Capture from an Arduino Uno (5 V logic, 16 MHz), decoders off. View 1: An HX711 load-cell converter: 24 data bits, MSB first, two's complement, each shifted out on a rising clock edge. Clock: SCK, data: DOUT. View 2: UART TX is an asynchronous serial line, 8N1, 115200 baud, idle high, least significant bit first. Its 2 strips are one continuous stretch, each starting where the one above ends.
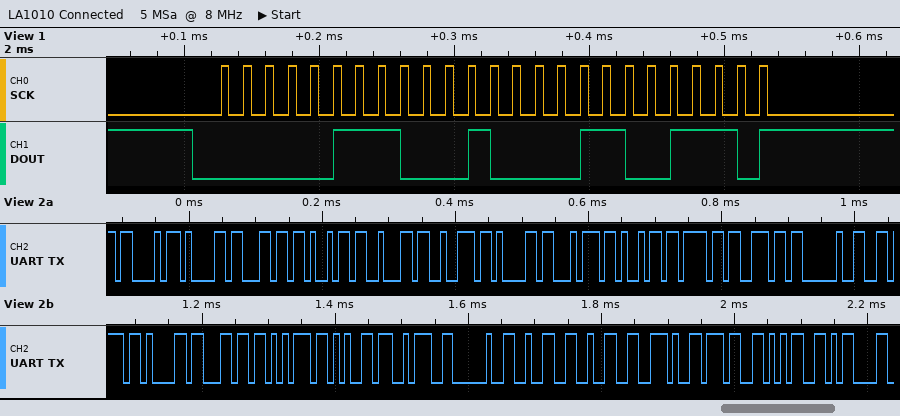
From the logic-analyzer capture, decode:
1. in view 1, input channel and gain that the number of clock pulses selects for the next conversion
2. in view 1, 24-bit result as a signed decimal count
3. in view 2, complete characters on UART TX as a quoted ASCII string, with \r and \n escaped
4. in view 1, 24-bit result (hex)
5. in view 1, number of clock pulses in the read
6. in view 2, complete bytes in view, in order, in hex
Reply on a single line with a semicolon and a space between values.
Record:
channel A, gain 128; 463054; "Calibration value: 22.75\r"; 0x0710CE; 25; 0x43 0x61 0x6C 0x69 0x62 0x72 0x61 0x74 0x69 0x6F 0x6E 0x20 0x76 0x61 0x6C 0x75 0x65 0x3A 0x20 0x32 0x32 0x2E 0x37 0x35 0x0D
